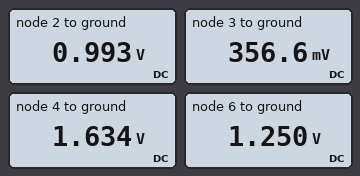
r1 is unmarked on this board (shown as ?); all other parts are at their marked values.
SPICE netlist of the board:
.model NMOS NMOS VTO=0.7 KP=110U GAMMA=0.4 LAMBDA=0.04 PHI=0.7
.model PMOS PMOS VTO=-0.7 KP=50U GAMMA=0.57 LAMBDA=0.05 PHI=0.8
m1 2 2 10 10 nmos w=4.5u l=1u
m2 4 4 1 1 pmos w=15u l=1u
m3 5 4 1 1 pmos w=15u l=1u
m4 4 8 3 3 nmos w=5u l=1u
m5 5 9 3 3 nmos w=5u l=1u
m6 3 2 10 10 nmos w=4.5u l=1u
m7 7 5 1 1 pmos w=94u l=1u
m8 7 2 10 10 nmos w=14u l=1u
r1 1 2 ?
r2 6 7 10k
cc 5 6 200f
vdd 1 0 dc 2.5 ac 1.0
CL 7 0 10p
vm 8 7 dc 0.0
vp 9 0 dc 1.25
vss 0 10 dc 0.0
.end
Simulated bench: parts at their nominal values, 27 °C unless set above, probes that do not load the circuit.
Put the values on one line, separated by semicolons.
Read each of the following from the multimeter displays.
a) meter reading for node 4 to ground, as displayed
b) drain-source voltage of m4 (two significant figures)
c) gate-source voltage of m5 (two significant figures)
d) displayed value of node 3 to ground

1.634 V; 1.3 V; 890 mV; 356.6 mV
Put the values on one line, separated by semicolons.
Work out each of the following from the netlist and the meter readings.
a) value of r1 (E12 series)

68 kΩ
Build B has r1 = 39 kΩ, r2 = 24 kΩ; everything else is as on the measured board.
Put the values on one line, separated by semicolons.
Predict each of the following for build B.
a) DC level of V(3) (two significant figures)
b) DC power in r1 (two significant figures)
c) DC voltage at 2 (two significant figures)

310 mV; 52 µW; 1.1 V
